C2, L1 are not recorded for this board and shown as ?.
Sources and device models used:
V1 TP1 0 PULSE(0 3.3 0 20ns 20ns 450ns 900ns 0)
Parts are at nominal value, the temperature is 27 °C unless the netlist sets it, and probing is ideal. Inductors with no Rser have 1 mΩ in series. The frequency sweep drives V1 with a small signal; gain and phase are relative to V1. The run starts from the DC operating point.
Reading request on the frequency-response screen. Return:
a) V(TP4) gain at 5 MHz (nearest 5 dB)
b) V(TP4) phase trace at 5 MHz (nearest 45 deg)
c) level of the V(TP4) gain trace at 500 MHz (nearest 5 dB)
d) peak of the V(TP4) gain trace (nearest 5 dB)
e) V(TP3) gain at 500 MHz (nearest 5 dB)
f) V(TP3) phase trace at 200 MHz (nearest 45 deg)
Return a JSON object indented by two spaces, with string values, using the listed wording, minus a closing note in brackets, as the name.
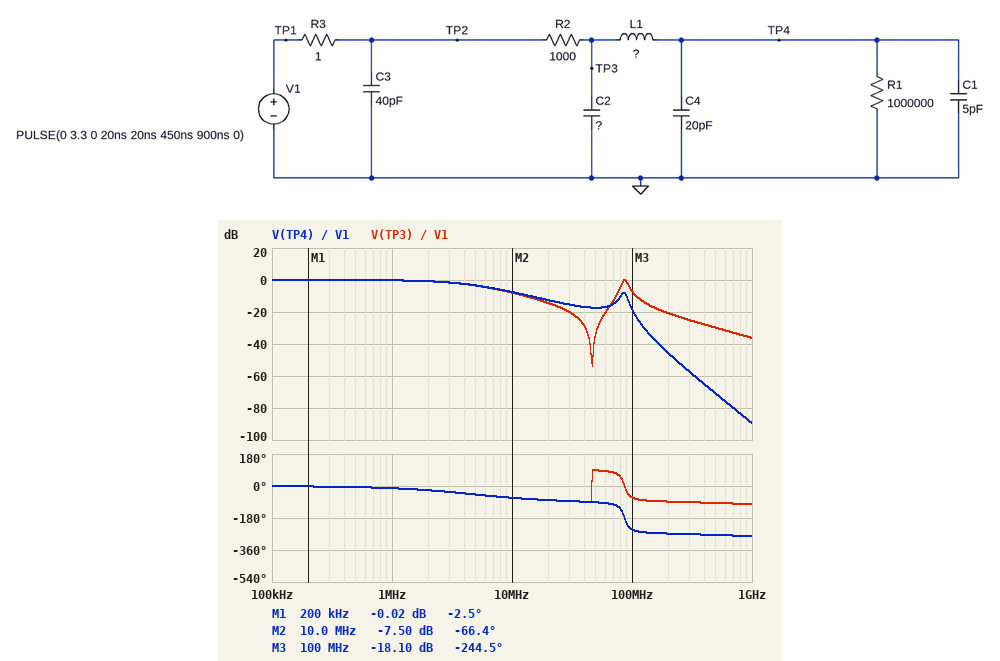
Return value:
{
  "V(TP4) gain at 5 MHz": "-5 dB",
  "V(TP4) phase trace at 5 MHz": "-45 deg",
  "level of the V(TP4) gain trace at 500 MHz": "-70 dB",
  "peak of the V(TP4) gain trace": "0 dB",
  "V(TP3) gain at 500 MHz": "-30 dB",
  "V(TP3) phase trace at 200 MHz": "-90 deg"
}
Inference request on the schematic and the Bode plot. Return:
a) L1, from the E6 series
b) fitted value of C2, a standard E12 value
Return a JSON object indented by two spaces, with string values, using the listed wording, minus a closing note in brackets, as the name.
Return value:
{
  "L1, from the E6 series": "470 nH",
  "fitted value of C2, a standard E12 value": "10 pF"
}
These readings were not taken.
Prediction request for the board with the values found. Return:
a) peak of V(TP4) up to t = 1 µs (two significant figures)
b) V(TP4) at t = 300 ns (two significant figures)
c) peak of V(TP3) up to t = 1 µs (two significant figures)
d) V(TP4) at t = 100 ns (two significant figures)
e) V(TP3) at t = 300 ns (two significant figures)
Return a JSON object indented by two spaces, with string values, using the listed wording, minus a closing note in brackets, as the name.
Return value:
{
  "peak of V(TP4) up to t = 1 µs": "3.3 V",
  "V(TP4) at t = 300 ns": "3.3 V",
  "peak of V(TP3) up to t = 1 µs": "3.3 V",
  "V(TP4) at t = 100 ns": "3.0 V",
  "V(TP3) at t = 300 ns": "3.3 V"
}
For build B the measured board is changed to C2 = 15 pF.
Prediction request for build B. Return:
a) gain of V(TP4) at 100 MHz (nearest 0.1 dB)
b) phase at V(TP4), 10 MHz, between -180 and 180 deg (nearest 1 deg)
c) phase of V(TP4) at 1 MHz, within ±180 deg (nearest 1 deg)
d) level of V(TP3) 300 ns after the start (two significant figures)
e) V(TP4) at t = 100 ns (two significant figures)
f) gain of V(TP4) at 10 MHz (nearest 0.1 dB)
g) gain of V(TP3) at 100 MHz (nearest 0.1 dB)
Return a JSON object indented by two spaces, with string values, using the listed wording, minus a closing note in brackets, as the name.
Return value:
{
  "gain of V(TP4) at 100 MHz": "-25.6 dB",
  "phase at V(TP4), 10 MHz, between -180 and 180 deg": "-69 deg",
  "phase of V(TP4) at 1 MHz, within ±180 deg": "-14 deg",
  "level of V(TP3) 300 ns after the start": "3.3 V",
  "V(TP4) at t = 100 ns": "2.9 V",
  "gain of V(TP4) at 10 MHz": "-8.5 dB",
  "gain of V(TP3) at 100 MHz": "-14.3 dB"
}
